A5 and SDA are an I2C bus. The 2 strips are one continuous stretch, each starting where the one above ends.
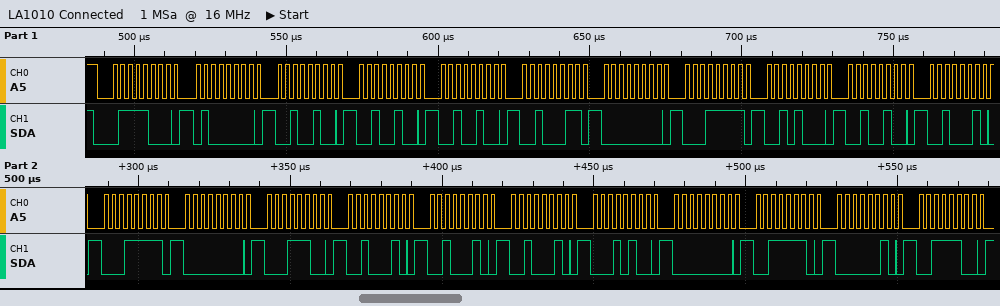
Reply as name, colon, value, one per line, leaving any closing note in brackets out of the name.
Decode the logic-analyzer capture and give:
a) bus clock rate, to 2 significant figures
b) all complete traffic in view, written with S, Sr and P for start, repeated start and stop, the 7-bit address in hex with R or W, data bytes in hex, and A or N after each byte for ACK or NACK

bus clock rate, to 2 significant figures: 400 kHz
all complete traffic in view, written with S, Sr and P for start, repeated start and stop, the 7-bit address in hex with R or W, data bytes in hex, and A or N after each byte for ACK or NACK: S 3CW A 40 A 24 A 24 A 24 A 23 A 00 A 1F A 28 A 24 A 22 A 1F A 00 A 1C A 22 A 22 A 22 A 14 A 00 A 3E A 02 A 3C A
